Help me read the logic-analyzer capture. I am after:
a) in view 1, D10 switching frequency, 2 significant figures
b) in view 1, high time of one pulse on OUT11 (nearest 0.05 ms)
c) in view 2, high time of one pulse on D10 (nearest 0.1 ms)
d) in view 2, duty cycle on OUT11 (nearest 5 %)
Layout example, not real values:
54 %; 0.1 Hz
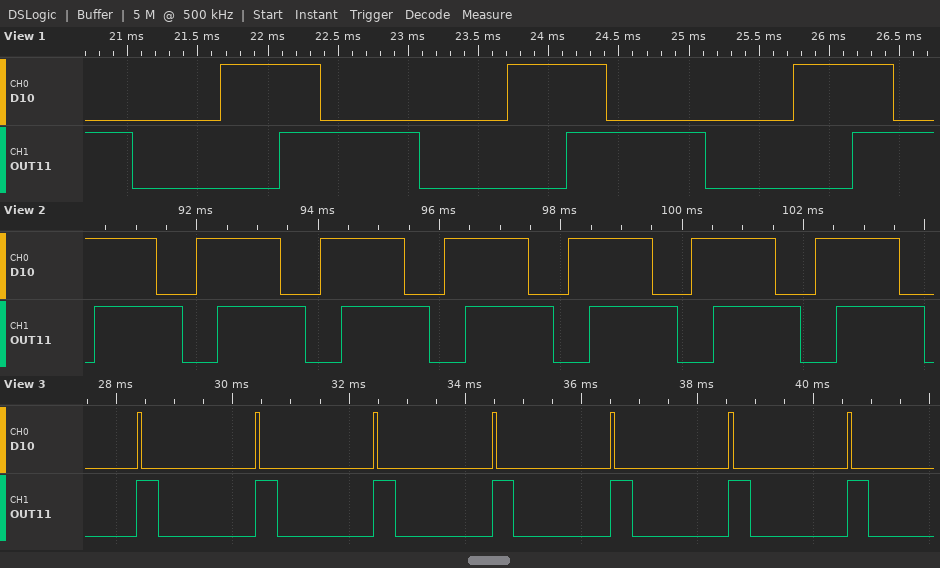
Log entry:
490 Hz; 1.00 ms; 1.4 ms; 70 %
